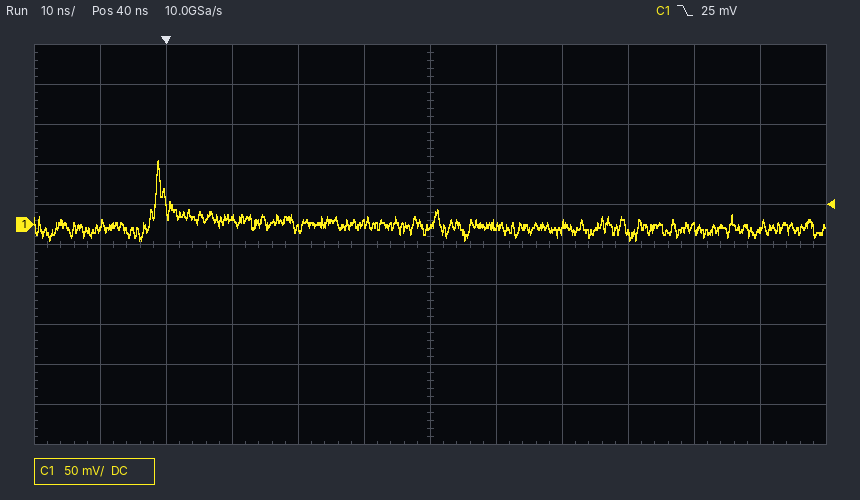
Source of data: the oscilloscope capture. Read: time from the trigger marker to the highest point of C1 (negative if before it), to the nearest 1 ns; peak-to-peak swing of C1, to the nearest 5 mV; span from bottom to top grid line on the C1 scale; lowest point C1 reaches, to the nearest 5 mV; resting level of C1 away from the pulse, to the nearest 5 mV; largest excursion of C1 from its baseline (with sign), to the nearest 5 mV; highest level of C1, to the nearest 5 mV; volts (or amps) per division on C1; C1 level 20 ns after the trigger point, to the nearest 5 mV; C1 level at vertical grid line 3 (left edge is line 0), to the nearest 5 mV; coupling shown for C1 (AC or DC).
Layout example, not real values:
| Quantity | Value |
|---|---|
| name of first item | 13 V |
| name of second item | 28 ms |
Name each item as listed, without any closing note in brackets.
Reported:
| Quantity | Value |
|---|---|
| time from the trigger marker to the highest point of C1 (negative if before it), to the nearest 1 ns | -1 ns |
| peak-to-peak swing of C1, to the nearest 5 mV | 100 mV |
| span from bottom to top grid line on the C1 scale | 500 mV |
| lowest point C1 reaches, to the nearest 5 mV | -20 mV |
| resting level of C1 away from the pulse, to the nearest 5 mV | 0 mV |
| largest excursion of C1 from its baseline (with sign), to the nearest 5 mV | +80 mV |
| highest level of C1, to the nearest 5 mV | 80 mV |
| volts (or amps) per division on C1 | 50 mV |
| C1 level 20 ns after the trigger point, to the nearest 5 mV | -5 mV |
| C1 level at vertical grid line 3 (left edge is line 0), to the nearest 5 mV | 10 mV |
| coupling shown for C1 | DC |
